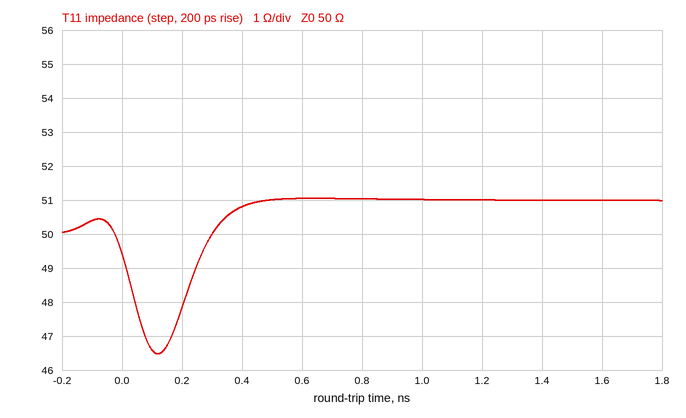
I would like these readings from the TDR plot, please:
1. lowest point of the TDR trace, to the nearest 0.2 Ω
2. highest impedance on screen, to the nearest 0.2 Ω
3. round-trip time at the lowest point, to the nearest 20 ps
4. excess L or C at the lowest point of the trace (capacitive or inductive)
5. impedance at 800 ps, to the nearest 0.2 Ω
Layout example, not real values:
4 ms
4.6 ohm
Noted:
46.4 Ω
51.0 Ω
120 ps
capacitive
51.0 Ω
